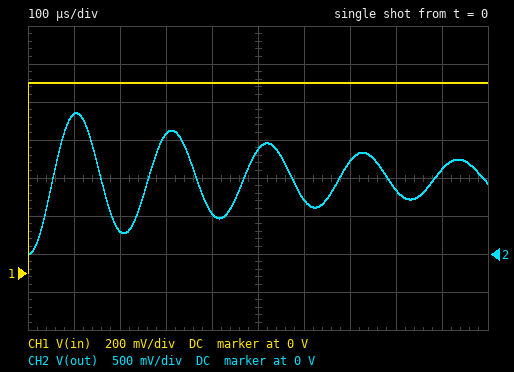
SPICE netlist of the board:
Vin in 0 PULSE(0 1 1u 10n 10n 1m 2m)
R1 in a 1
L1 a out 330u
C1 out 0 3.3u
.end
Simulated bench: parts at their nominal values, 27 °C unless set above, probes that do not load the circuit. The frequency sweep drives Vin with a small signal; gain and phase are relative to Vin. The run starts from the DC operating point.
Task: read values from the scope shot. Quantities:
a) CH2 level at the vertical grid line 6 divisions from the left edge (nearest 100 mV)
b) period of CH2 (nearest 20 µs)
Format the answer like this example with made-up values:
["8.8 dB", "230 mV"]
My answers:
["700 mV", "200 µs"]
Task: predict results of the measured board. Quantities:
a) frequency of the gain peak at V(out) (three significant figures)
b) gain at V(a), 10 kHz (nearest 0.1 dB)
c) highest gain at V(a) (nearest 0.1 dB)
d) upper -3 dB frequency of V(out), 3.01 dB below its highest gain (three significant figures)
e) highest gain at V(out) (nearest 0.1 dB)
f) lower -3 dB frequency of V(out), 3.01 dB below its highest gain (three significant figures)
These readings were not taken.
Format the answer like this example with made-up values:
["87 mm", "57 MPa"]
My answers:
["4.81 kHz", "0 dB", "0 dB", "5.05 kHz", "20.0 dB", "4.56 kHz"]
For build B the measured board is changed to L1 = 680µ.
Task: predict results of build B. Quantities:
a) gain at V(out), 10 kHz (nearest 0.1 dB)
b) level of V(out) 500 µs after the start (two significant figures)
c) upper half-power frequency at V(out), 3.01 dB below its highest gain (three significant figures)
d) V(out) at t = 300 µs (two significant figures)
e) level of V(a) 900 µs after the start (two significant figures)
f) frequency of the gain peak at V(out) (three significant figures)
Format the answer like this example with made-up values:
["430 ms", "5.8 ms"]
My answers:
["-17.9 dB", "1.3 V", "3.47 kHz", "200 mV", "1.0 V", "3.36 kHz"]
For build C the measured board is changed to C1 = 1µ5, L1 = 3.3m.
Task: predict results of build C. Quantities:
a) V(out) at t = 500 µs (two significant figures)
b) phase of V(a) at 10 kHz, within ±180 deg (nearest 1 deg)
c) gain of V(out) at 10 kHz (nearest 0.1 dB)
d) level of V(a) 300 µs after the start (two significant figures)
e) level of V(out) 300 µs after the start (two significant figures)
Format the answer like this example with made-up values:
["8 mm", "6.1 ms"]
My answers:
["350 mV", "0 deg", "-25.4 dB", "1.0 V", "1.4 V"]
